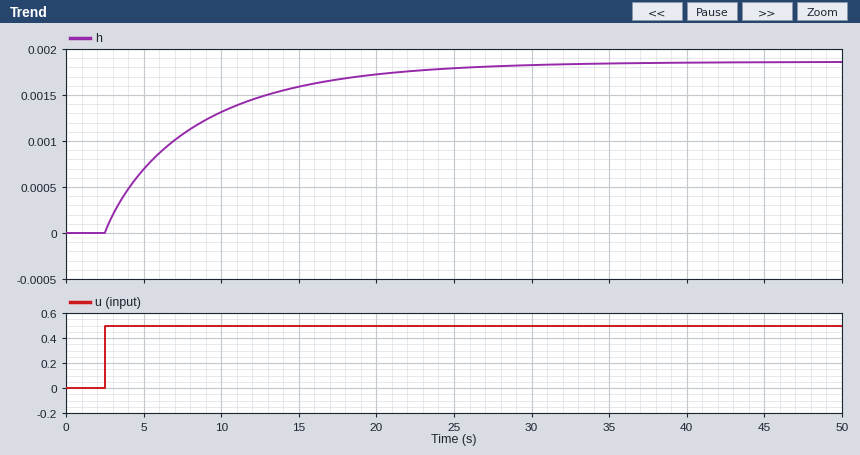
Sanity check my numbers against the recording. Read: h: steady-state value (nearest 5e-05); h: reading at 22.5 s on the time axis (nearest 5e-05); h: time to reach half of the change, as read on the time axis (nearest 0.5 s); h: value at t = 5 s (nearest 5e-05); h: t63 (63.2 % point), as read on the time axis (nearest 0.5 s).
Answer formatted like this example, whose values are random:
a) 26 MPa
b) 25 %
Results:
a) 0.00185
b) 0.00175
c) 6.5 s
d) 0.00070
e) 8.5 s
